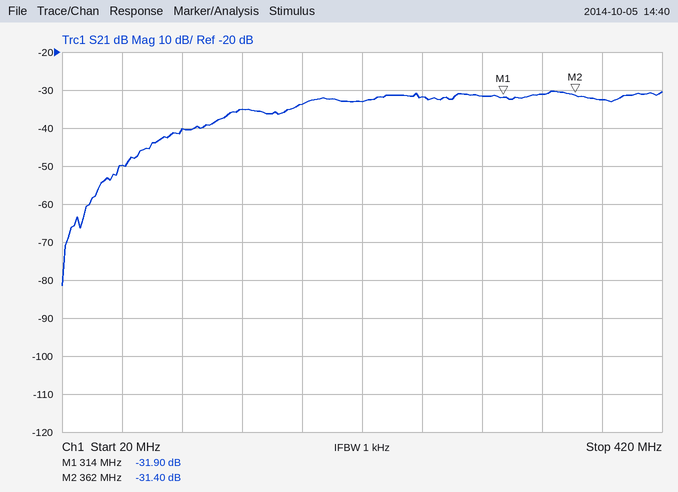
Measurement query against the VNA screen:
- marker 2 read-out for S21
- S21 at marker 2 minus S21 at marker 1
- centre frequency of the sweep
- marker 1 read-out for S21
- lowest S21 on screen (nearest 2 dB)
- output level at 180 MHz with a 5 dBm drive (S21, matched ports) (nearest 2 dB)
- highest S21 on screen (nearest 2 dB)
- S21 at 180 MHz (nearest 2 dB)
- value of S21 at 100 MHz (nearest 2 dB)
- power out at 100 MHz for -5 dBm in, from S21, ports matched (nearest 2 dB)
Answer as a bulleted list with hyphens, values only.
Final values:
- -31.40 dB
- 0.50 dB
- 220 MHz
- -31.90 dB
- -82 dB
- -28 dBm
- -30 dB
- -34 dB
- -40 dB
- -46 dBm
